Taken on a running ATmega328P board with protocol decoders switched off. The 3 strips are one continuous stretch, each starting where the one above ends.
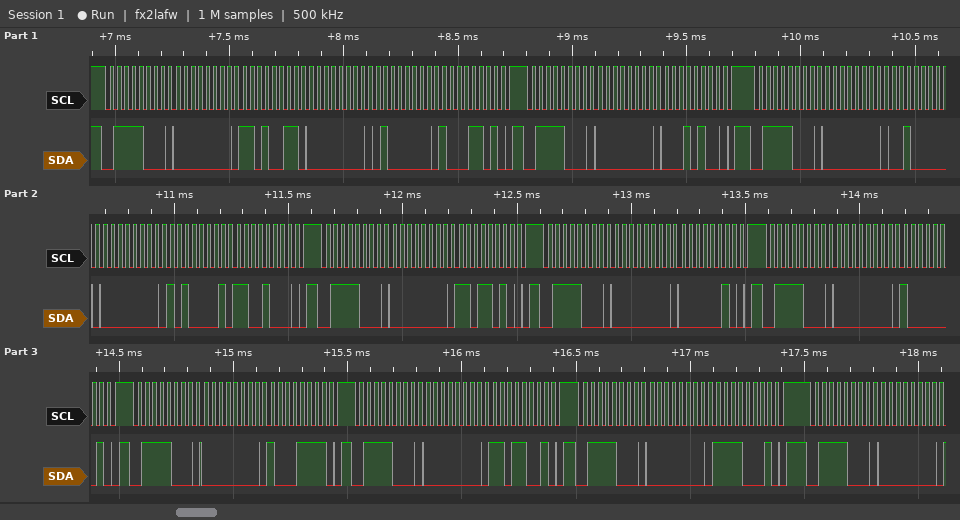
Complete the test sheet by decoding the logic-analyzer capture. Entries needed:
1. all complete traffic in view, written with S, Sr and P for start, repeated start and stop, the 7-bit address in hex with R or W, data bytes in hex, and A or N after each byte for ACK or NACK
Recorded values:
S 3CW A 00 A D3 A 00 A 40 A 8D A P S 3CW A 00 A 14 A P S 3CW A 00 A 20 A 00 A A1 A C8 A P S 3CW A 00 A DA A P S 3CW A 00 A 02 A P S 3CW A 00 A 81 A P S 3CW A 00 A 8F A P S 3CW A 00 A D9 A P S 3CW A 00 A F1 A P S 3CW A 00 A
